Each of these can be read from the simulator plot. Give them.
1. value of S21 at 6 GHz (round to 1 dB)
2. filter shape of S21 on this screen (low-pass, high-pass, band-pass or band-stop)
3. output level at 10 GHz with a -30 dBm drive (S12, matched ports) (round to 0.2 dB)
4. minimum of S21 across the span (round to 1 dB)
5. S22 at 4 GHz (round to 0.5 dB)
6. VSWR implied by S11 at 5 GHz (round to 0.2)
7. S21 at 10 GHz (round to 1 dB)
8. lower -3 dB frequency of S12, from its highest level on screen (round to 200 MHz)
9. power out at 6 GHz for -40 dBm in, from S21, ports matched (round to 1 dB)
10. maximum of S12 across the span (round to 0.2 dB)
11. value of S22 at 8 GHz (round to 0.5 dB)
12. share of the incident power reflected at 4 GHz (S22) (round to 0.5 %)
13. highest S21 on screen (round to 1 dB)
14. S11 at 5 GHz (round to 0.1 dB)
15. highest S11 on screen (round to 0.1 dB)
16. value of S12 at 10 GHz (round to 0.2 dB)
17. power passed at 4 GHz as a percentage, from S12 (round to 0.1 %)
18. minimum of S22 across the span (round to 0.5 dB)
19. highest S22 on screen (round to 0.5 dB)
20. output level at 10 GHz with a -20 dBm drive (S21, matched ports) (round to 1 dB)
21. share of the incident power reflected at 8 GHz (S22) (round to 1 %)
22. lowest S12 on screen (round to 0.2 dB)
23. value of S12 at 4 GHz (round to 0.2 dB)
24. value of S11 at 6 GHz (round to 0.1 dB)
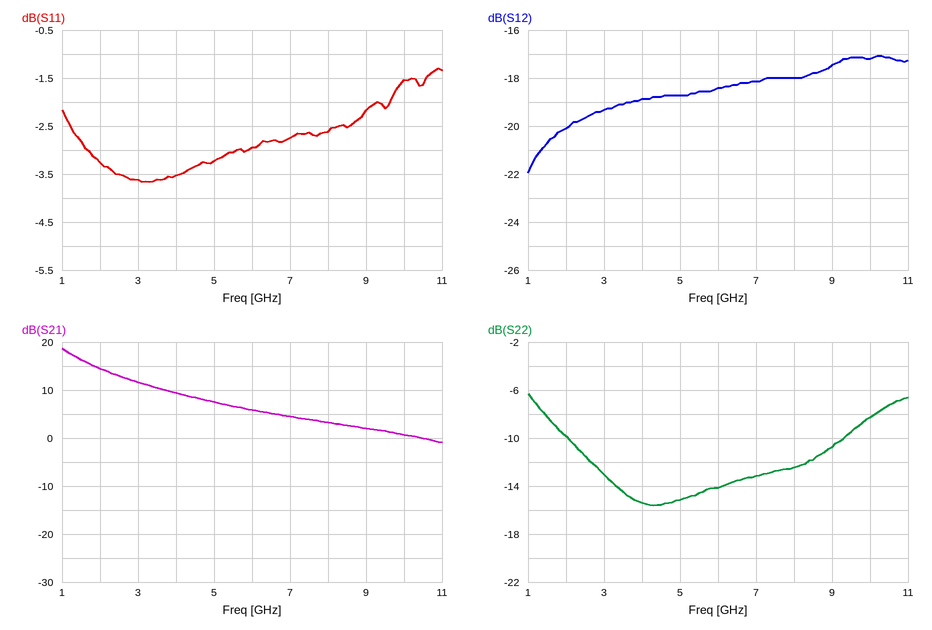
6 dB
low-pass
-47.2 dBm
-1 dB
-15.5 dB
5.4
1 dB
2.0 GHz
-34 dBm
-17.0 dB
-12.5 dB
3.0 %
19 dB
-3.2 dB
-1.3 dB
-17.2 dB
1.3 %
-15.5 dB
-6.5 dB
-19 dBm
6 %
-22.0 dB
-18.8 dB
-2.9 dB
